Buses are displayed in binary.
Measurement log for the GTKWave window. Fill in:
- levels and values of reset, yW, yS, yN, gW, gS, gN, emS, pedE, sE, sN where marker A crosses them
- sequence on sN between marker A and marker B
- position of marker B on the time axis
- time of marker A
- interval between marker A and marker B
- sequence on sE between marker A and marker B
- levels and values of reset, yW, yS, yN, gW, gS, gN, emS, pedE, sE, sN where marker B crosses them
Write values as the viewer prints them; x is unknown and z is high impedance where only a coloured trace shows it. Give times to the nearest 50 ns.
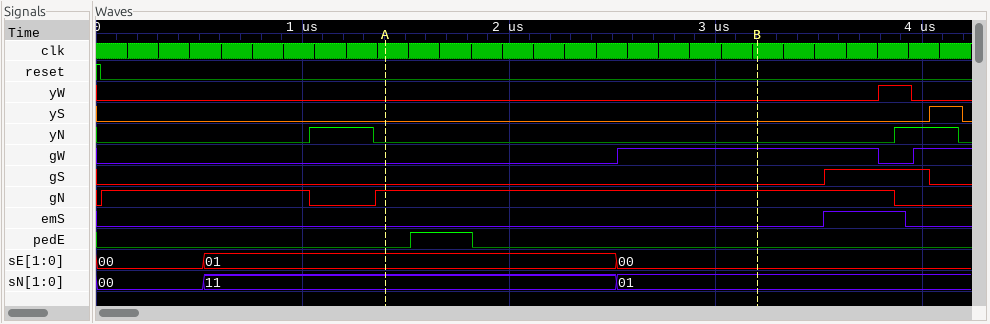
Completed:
reset=0, yW=0, yS=0, yN=0, gW=0, gS=0, gN=1, emS=0, pedE=0, sE=01, sN=11
11, 01
3200 ns
1400 ns
1800 ns
01, 00
reset=0, yW=0, yS=0, yN=0, gW=1, gS=0, gN=1, emS=0, pedE=0, sE=00, sN=01
